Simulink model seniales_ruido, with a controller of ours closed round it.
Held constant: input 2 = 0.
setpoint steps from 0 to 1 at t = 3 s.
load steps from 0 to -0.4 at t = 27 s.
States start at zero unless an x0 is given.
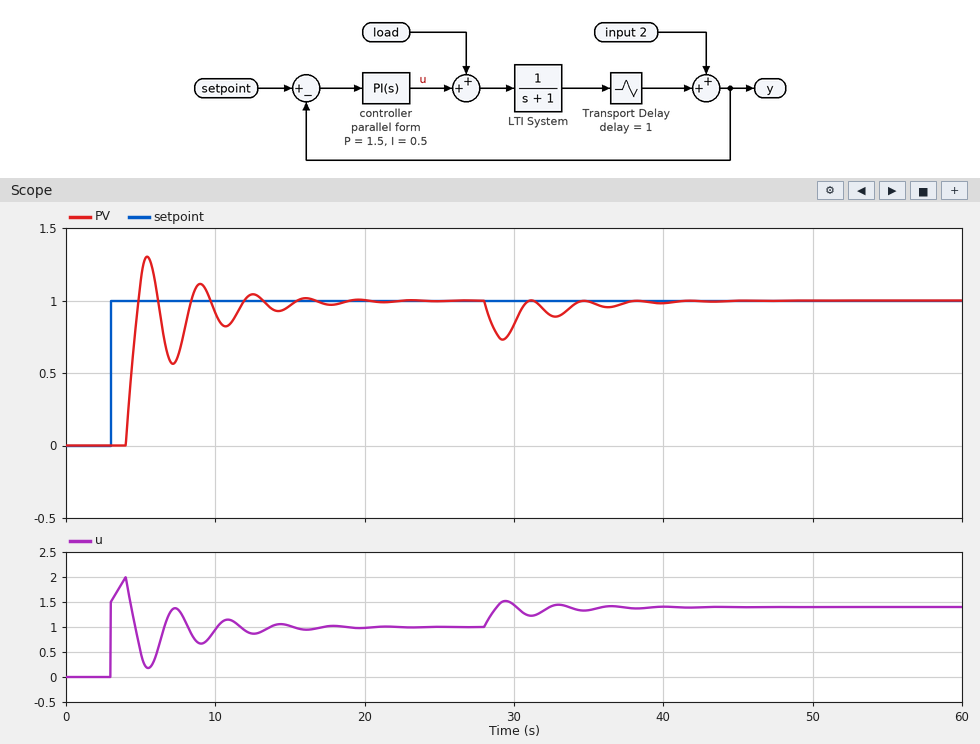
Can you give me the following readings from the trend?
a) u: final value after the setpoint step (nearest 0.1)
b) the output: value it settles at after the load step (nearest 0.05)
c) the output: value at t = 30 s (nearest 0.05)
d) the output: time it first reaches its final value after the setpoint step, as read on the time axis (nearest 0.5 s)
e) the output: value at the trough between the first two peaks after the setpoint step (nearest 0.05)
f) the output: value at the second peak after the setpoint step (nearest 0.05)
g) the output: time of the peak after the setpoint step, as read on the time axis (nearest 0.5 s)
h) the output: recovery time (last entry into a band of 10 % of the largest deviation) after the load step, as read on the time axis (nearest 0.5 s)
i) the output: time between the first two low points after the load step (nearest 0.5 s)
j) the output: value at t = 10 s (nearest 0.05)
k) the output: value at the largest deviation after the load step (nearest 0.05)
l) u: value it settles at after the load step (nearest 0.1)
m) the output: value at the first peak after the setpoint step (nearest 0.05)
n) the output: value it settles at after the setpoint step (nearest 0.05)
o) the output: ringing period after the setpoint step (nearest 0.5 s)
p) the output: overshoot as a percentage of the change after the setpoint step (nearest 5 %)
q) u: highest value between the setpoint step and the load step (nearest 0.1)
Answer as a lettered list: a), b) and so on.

a) 1.0
b) 1.00
c) 0.85
d) 5.0 s
e) 0.55
f) 1.10
g) 5.5 s
h) 37.0 s
i) 3.5 s
j) 0.90
k) 0.75
l) 1.4
m) 1.30
n) 1.00
o) 3.5 s
p) 30 %
q) 2.0
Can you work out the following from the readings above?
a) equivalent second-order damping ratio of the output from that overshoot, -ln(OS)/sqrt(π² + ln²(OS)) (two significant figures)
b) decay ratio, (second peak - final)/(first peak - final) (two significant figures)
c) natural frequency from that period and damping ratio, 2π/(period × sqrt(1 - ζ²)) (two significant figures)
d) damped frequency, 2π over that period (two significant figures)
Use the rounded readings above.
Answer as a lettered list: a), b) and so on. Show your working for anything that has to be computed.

a) ln(0.3) = -1.204; 1.204 / sqrt(9.870 + 1.450) = 0.36
b) (1.1 - 1) / (1.3 - 1) = 0.33
c) 2π / (3.5 × sqrt(1 - 0.36²)) = 1.9 rad/s
d) 2π / 3.5 = 1.8 rad/s
